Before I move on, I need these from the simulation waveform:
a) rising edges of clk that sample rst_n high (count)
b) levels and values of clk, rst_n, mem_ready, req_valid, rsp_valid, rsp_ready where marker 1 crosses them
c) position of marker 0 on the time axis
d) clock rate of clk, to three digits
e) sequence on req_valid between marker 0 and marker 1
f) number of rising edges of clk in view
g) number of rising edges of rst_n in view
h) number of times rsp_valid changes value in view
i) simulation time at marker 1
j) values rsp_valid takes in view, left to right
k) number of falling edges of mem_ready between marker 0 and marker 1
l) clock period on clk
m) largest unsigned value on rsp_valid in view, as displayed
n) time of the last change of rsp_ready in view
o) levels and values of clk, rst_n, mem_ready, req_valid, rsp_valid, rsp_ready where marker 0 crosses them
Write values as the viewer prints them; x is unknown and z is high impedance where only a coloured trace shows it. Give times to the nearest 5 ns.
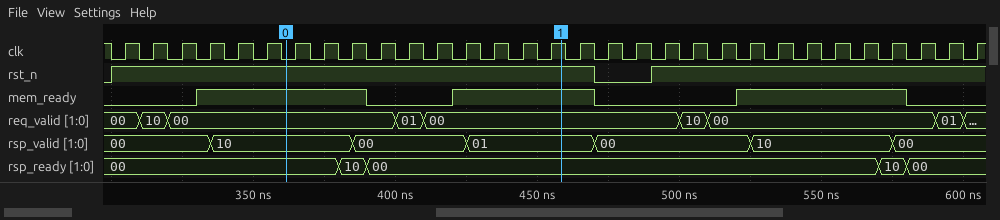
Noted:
29
clk=1, rst_n=1, mem_ready=1, req_valid=00, rsp_valid=01, rsp_ready=00
360 ns
100 MHz
00, 01, 00
31
2
6
460 ns
00, 10, 00, 01, 00, 10, 00
1
10 ns
10
580 ns
clk=0, rst_n=1, mem_ready=1, req_valid=00, rsp_valid=10, rsp_ready=00
